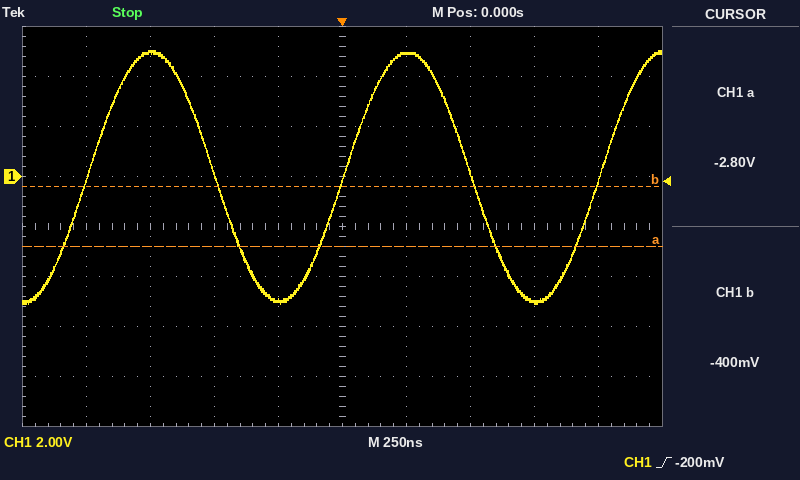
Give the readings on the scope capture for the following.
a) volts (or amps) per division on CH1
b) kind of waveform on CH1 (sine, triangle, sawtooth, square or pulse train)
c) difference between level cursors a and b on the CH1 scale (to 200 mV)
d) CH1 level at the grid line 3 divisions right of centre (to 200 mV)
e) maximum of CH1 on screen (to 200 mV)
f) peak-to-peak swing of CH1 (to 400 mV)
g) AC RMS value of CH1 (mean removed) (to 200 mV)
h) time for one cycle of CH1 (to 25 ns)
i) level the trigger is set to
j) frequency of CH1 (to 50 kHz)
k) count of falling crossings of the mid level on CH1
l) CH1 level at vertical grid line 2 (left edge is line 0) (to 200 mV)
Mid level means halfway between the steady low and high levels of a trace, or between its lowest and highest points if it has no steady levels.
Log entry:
2 V
sine
2.4 V
-5.0 V
5.0 V
10.0 V
3.6 V
1.000 µs
-200 mV
1.00 MHz
2
5.0 V
